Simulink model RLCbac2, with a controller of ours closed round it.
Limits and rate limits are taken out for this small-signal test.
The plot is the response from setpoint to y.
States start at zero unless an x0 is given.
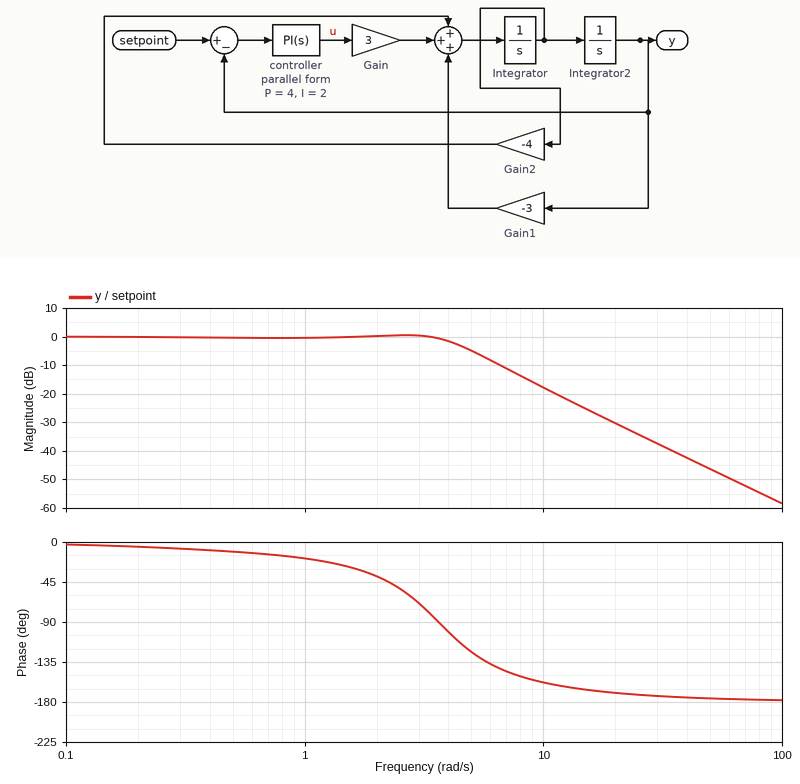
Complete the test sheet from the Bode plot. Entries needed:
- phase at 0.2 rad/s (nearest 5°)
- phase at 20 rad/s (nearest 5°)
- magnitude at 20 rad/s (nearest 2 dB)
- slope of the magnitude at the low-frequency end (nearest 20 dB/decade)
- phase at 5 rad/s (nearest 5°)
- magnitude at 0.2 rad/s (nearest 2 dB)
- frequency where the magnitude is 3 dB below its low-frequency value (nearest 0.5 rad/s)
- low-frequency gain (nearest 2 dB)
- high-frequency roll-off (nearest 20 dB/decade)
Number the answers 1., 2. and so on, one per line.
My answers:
1. -5°
2. -170°
3. -30 dB
4. 0 dB/decade
5. -125°
6. 0 dB
7. 4.5 rad/s
8. 0 dB
9. -40 dB/decade
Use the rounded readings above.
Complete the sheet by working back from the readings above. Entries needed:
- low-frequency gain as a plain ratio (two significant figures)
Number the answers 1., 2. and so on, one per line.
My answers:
1. 1.0
